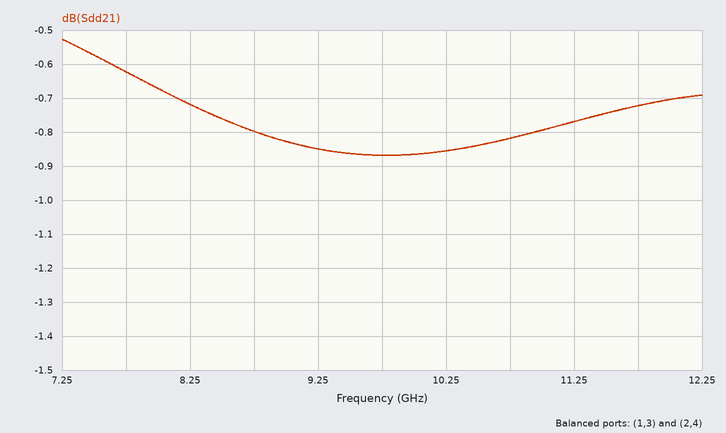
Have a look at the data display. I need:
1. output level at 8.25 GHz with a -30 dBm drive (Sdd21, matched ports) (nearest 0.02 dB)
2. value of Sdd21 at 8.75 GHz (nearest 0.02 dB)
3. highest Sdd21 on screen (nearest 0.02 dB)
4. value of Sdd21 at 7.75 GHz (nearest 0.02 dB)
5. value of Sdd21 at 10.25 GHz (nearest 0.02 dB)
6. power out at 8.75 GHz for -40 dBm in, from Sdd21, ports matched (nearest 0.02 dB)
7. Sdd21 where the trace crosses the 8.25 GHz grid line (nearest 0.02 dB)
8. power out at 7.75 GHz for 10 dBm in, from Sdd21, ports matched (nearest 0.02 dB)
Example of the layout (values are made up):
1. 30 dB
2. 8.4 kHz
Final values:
1. -30.72 dBm
2. -0.80 dB
3. -0.52 dB
4. -0.62 dB
5. -0.86 dB
6. -40.80 dBm
7. -0.72 dB
8. 9.38 dBm
